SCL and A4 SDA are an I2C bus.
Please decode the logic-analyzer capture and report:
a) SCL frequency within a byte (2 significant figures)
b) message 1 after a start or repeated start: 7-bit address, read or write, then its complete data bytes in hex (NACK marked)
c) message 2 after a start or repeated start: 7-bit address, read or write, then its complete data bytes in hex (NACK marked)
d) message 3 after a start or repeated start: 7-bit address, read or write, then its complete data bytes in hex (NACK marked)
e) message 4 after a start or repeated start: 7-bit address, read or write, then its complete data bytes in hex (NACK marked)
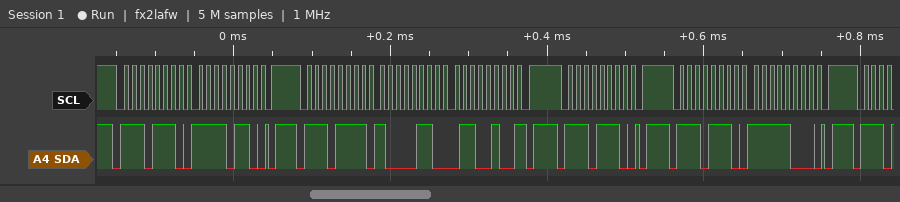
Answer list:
100 kHz
0x77 write: F6
0x77 read: 86 64 NACK
0x77 write
0x77 write: F8
